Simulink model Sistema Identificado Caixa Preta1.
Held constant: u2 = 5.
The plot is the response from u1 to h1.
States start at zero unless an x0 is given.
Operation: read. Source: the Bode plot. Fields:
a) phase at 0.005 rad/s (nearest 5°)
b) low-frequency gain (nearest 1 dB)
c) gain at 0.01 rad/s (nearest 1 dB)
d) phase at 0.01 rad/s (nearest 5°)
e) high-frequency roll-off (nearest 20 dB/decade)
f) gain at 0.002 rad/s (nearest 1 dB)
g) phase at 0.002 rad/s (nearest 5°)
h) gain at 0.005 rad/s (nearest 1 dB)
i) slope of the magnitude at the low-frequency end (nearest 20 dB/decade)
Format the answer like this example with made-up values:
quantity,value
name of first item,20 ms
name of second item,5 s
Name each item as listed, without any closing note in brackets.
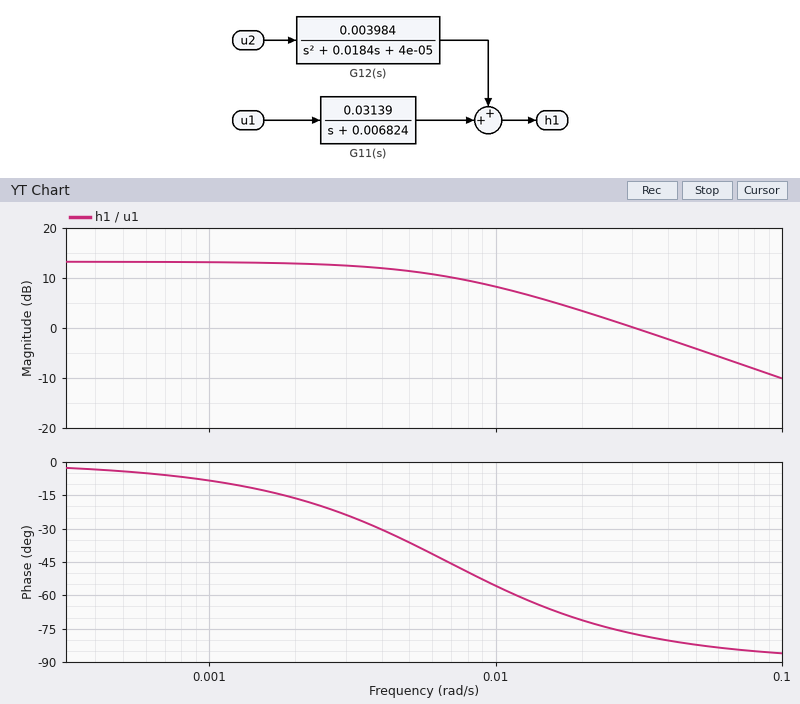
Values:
quantity,value
phase at 0.005 rad/s,-35°
low-frequency gain,13 dB
gain at 0.01 rad/s,8 dB
phase at 0.01 rad/s,-55°
high-frequency roll-off,-20 dB/decade
gain at 0.002 rad/s,13 dB
phase at 0.002 rad/s,-15°
gain at 0.005 rad/s,11 dB
slope of the magnitude at the low-frequency end,0 dB/decade
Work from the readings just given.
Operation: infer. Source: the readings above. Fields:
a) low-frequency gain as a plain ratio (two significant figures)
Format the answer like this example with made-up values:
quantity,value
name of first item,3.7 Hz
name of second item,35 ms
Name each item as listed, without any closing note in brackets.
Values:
quantity,value
low-frequency gain as a plain ratio,4.5
